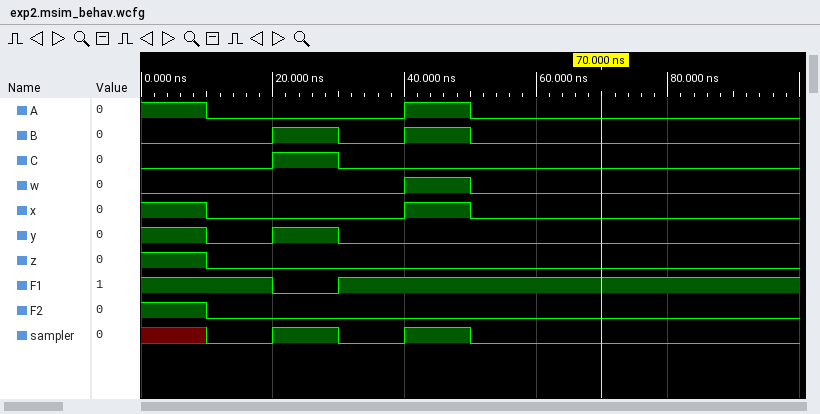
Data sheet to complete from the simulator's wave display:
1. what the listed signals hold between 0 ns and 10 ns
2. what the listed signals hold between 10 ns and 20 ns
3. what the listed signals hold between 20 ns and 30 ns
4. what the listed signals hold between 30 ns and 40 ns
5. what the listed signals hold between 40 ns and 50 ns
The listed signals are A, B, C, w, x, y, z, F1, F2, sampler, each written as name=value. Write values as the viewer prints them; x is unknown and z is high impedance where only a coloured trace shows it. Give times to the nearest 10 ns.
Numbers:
A=1, B=0, C=0, w=0, x=1, y=1, z=1, F1=1, F2=1, sampler=x
A=0, B=0, C=0, w=0, x=0, y=0, z=0, F1=1, F2=0, sampler=0
A=0, B=1, C=1, w=0, x=0, y=1, z=0, F1=0, F2=0, sampler=1
A=0, B=0, C=0, w=0, x=0, y=0, z=0, F1=1, F2=0, sampler=0
A=1, B=1, C=0, w=1, x=1, y=0, z=0, F1=1, F2=0, sampler=1
